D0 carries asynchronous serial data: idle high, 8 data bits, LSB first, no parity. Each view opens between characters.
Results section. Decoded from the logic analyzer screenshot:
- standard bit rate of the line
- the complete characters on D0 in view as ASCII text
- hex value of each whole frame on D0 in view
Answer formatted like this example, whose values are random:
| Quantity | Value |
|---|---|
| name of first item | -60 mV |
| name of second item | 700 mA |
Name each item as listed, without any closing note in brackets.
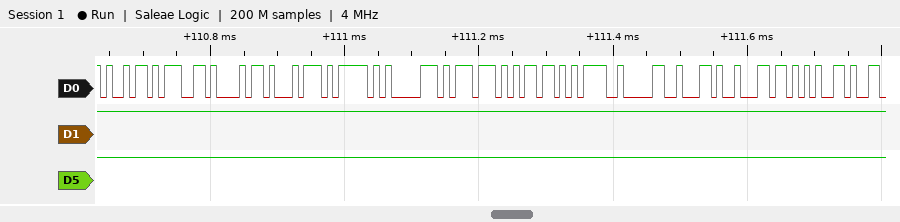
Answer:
| Quantity | Value |
|---|---|
| standard bit rate of the line | 115200 baud |
| the complete characters on D0 in view as ASCII text | "ight_pwm=0,le" |
| hex value of each whole frame on D0 in view | 69, 67, 68, 74, 5F, 70, 77, 6D, 3D, 30, 2C, 6C, 65 |
